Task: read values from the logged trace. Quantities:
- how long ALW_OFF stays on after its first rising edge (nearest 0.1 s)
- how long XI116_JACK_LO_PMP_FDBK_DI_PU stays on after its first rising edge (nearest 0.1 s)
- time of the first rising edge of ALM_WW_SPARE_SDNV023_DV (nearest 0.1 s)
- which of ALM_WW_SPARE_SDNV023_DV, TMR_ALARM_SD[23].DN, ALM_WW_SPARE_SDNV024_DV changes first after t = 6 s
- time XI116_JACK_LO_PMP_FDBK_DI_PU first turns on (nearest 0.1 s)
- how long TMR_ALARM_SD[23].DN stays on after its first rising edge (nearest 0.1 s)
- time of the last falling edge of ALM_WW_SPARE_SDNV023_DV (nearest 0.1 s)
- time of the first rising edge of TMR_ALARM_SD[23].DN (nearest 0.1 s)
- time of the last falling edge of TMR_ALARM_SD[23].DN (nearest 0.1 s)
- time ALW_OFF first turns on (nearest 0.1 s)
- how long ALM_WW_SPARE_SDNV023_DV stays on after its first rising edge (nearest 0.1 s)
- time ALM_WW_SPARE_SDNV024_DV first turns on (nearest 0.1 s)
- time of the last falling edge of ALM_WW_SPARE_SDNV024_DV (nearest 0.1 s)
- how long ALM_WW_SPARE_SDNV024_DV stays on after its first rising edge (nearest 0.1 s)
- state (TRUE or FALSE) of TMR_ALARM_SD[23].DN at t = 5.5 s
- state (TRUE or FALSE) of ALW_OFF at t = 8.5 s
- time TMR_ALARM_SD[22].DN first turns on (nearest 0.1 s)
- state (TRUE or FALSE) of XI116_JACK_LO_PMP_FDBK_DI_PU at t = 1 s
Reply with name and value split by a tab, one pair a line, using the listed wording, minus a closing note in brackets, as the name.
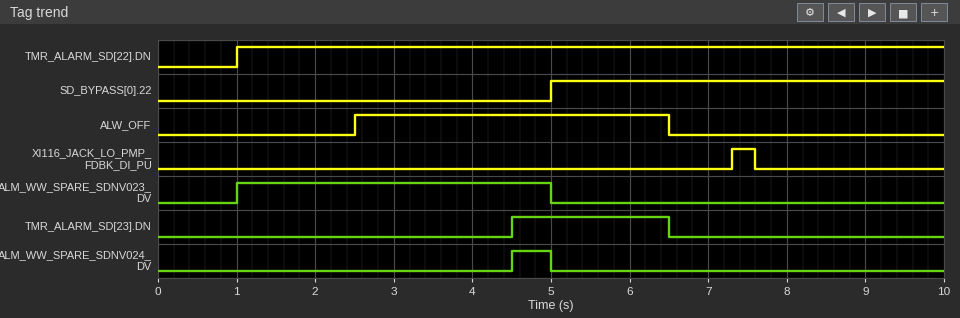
how long ALW_OFF stays on after its first rising edge	4.0 s
how long XI116_JACK_LO_PMP_FDBK_DI_PU stays on after its first rising edge	0.3 s
time of the first rising edge of ALM_WW_SPARE_SDNV023_DV	1.0 s
which of ALM_WW_SPARE_SDNV023_DV, TMR_ALARM_SD[23].DN, ALM_WW_SPARE_SDNV024_DV changes first after t = 6 s	TMR_ALARM_SD[23].DN
time XI116_JACK_LO_PMP_FDBK_DI_PU first turns on	7.3 s
how long TMR_ALARM_SD[23].DN stays on after its first rising edge	2.0 s
time of the last falling edge of ALM_WW_SPARE_SDNV023_DV	5.0 s
time of the first rising edge of TMR_ALARM_SD[23].DN	4.5 s
time of the last falling edge of TMR_ALARM_SD[23].DN	6.5 s
time ALW_OFF first turns on	2.5 s
how long ALM_WW_SPARE_SDNV023_DV stays on after its first rising edge	4.0 s
time ALM_WW_SPARE_SDNV024_DV first turns on	4.5 s
time of the last falling edge of ALM_WW_SPARE_SDNV024_DV	5.0 s
how long ALM_WW_SPARE_SDNV024_DV stays on after its first rising edge	0.5 s
state (TRUE or FALSE) of TMR_ALARM_SD[23].DN at t = 5.5 s	TRUE
state (TRUE or FALSE) of ALW_OFF at t = 8.5 s	FALSE
time TMR_ALARM_SD[22].DN first turns on	1.0 s
state (TRUE or FALSE) of XI116_JACK_LO_PMP_FDBK_DI_PU at t = 1 s	FALSE
